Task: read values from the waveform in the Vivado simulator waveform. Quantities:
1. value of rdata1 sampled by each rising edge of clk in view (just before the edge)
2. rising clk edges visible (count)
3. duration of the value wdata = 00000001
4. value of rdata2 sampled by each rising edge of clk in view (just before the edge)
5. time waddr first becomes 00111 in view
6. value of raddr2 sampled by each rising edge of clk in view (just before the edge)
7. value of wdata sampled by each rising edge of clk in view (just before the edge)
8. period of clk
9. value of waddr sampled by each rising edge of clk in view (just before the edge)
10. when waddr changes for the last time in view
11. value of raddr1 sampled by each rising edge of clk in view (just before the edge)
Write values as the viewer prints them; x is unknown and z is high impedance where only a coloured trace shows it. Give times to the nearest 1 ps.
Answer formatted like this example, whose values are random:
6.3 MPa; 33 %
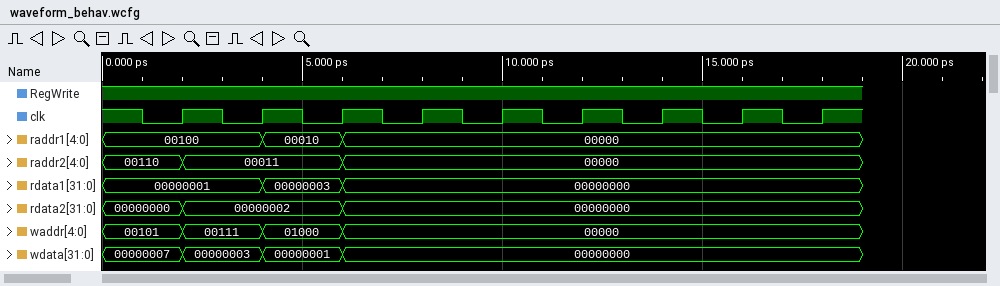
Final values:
00000001, 00000001, 00000003, 00000000, 00000000, 00000000, 00000000, 00000000, 00000000; 9; 2 ps; 00000000, 00000002, 00000002, 00000000, 00000000, 00000000, 00000000, 00000000, 00000000; 2 ps; 00110, 00011, 00011, 00000, 00000, 00000, 00000, 00000, 00000; 00000007, 00000003, 00000001, 00000000, 00000000, 00000000, 00000000, 00000000, 00000000; 2 ps; 00101, 00111, 01000, 00000, 00000, 00000, 00000, 00000, 00000; 6 ps; 00100, 00100, 00010, 00000, 00000, 00000, 00000, 00000, 00000
